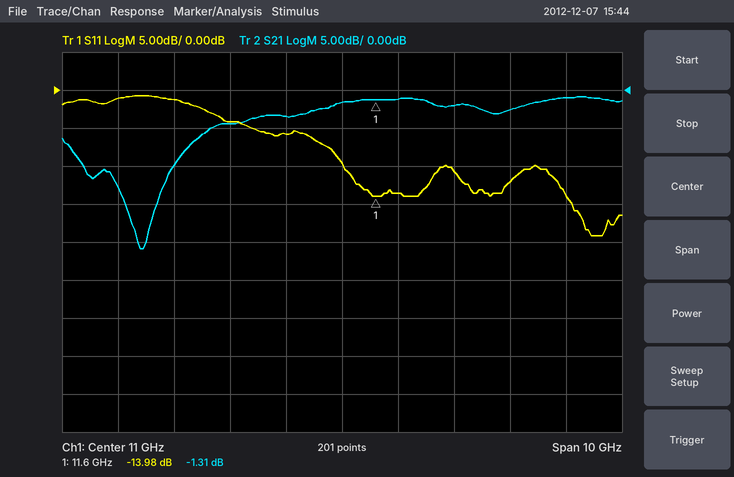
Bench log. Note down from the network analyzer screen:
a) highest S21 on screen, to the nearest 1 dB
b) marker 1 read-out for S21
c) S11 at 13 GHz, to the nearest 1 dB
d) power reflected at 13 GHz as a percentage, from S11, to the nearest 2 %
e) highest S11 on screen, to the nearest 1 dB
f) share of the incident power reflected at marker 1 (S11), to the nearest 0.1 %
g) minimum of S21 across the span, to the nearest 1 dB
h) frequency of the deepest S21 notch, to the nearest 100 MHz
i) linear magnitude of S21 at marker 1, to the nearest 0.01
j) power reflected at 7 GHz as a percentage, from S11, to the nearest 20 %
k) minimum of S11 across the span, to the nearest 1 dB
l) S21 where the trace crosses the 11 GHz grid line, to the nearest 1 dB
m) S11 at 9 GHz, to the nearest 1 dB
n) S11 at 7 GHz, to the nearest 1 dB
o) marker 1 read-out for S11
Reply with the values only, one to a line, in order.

-1 dB
-1.31 dB
-11 dB
8 %
-1 dB
4.0 %
-21 dB
7.4 GHz
0.86
80 %
-19 dB
-2 dB
-4 dB
-1 dB
-13.98 dB
